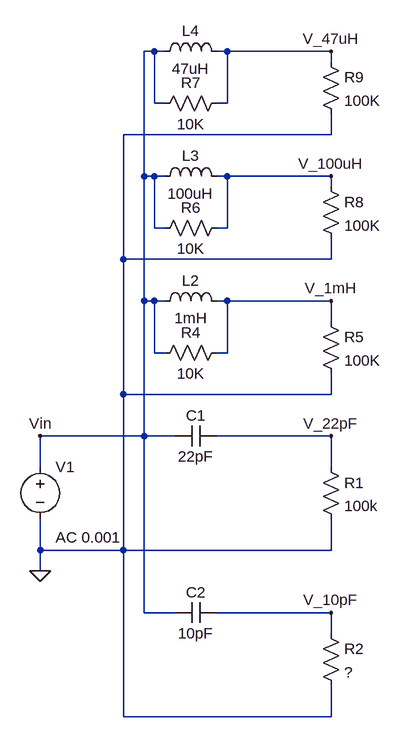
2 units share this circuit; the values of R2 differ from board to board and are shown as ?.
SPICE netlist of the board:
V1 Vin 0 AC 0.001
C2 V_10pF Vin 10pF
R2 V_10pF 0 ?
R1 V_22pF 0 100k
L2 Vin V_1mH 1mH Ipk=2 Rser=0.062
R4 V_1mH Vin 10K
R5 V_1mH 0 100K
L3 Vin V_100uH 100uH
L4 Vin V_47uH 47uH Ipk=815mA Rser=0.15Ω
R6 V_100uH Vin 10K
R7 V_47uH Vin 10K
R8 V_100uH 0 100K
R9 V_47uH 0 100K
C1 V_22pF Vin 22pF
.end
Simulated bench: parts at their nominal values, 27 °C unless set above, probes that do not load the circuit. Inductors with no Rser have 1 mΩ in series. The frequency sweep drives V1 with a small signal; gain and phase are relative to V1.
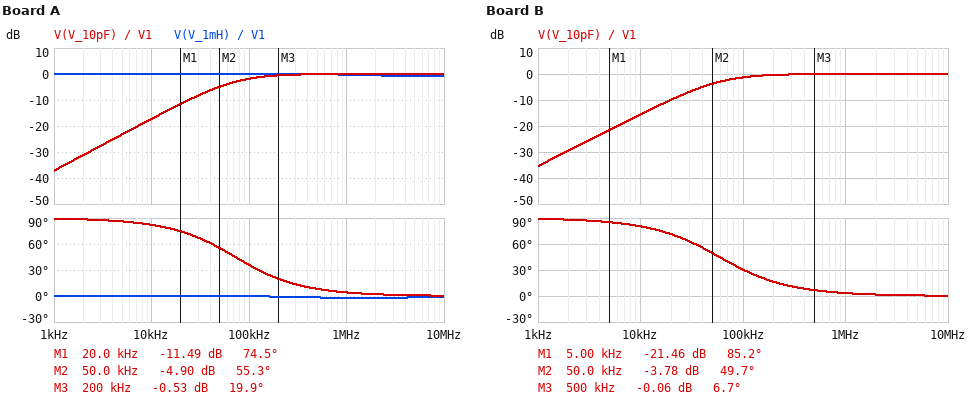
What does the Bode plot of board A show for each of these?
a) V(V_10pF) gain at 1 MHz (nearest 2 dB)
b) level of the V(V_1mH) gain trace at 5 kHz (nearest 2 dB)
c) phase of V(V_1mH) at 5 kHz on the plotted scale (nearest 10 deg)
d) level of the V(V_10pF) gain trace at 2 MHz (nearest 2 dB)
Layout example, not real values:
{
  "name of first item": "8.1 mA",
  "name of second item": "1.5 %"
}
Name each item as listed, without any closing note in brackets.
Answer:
{
  "V(V_10pF) gain at 1 MHz": "0 dB",
  "level of the V(V_1mH) gain trace at 5 kHz": "0 dB",
  "phase of V(V_1mH) at 5 kHz on the plotted scale": "0 deg",
  "level of the V(V_10pF) gain trace at 2 MHz": "0 dB"
}
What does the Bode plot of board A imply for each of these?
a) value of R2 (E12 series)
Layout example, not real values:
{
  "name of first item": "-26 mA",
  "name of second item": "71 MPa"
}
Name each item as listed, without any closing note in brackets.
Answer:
{
  "value of R2": "220 kΩ"
}
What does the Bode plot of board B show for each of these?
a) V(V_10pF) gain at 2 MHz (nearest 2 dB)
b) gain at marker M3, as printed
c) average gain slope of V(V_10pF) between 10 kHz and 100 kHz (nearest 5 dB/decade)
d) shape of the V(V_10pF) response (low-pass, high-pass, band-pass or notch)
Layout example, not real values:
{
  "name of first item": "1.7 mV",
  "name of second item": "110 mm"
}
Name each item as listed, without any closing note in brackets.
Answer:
{
  "V(V_10pF) gain at 2 MHz": "0 dB",
  "gain at marker M3, as printed": "-0.06 dB",
  "average gain slope of V(V_10pF) between 10 kHz and 100 kHz": "15 dB/decade",
  "shape of the V(V_10pF) response": "high-pass"
}
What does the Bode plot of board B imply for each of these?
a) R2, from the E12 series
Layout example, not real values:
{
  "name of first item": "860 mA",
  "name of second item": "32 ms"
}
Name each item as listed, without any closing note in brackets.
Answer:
{
  "R2, from the E12 series": "270 kΩ"
}
